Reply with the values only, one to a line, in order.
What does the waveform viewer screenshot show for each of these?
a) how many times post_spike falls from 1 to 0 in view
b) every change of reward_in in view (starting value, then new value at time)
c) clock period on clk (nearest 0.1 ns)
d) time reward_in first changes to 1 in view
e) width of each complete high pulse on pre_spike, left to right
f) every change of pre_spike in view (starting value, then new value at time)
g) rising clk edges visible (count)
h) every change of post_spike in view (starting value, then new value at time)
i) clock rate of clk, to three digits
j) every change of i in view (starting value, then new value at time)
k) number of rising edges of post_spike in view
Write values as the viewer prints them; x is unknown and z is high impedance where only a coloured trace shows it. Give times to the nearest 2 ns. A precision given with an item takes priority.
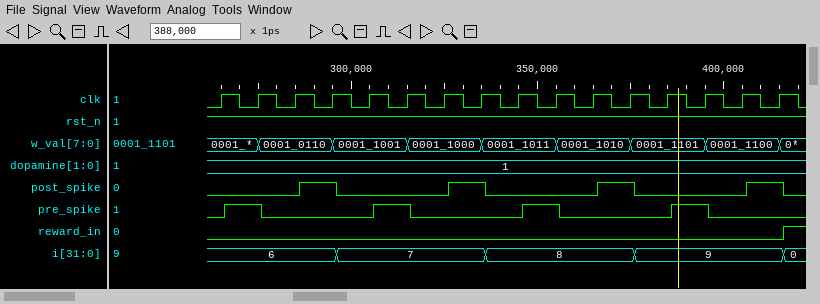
4
0, 1 at 416 ns
10 ns
416 ns
10 ns, 10 ns, 10 ns, 10 ns
0, 1 at 266 ns, 0 at 276 ns, 1 at 306 ns, 0 at 316 ns, 1 at 346 ns, 0 at 356 ns, 1 at 386 ns, 0 at 396 ns
16
0, 1 at 286 ns, 0 at 296 ns, 1 at 326 ns, 0 at 336 ns, 1 at 366 ns, 0 at 376 ns, 1 at 406 ns, 0 at 416 ns
100 MHz
6, 7 at 296 ns, 8 at 336 ns, 9 at 376 ns, 0 at 416 ns
4
